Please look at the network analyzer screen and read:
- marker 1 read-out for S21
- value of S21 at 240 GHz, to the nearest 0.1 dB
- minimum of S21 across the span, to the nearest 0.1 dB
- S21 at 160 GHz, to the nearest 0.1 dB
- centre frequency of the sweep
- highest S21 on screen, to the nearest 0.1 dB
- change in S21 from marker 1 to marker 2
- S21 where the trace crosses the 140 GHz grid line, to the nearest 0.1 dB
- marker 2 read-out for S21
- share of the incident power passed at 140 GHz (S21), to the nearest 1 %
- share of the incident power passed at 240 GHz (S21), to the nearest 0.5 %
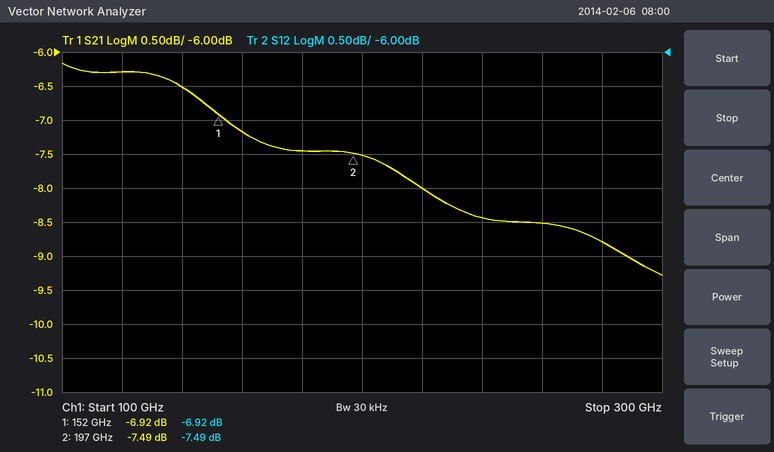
-6.92 dB
-8.4 dB
-9.3 dB
-7.2 dB
200 GHz
-6.2 dB
-0.57 dB
-6.5 dB
-7.49 dB
22 %
14.5 %
